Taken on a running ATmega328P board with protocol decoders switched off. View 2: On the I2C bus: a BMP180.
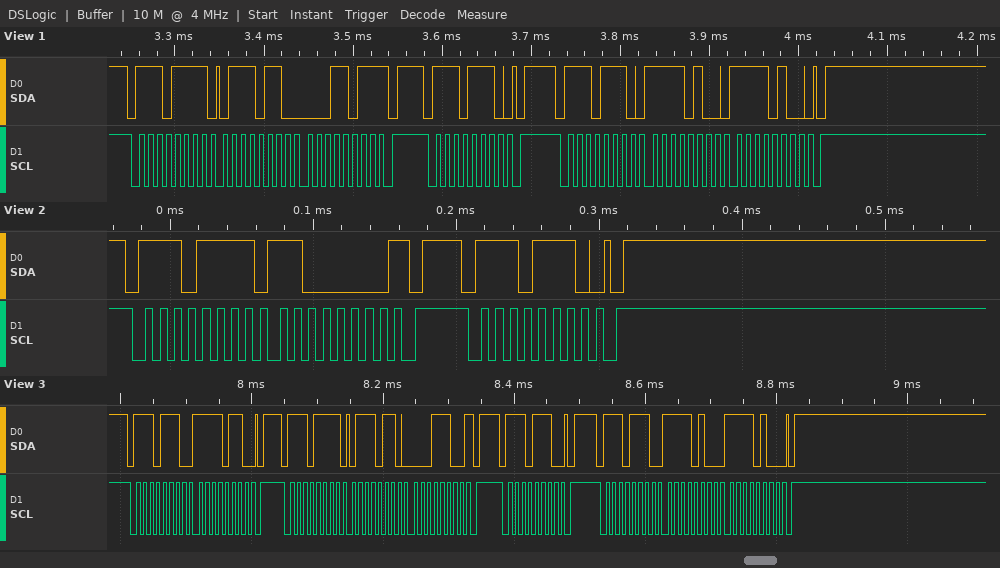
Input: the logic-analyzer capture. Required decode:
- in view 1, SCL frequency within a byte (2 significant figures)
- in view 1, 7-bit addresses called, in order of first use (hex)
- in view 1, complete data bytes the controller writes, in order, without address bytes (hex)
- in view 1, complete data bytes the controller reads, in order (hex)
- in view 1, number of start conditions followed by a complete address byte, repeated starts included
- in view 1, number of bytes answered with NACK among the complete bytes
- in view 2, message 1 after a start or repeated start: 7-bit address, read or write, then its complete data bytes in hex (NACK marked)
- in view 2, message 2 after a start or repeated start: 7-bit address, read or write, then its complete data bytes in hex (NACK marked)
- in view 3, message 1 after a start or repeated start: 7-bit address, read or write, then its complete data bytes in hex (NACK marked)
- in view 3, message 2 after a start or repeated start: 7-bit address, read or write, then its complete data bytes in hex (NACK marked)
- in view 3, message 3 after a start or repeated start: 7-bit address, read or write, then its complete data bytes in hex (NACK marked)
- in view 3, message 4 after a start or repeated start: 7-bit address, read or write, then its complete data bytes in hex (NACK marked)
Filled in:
100 kHz
0x77
F4 F4
76 1B
3
1
0x77 read: C0 NACK
0x77 write
0x77 write: F6
0x77 read: 76 1C NACK
0x77 write
0x77 write: F4 F4
